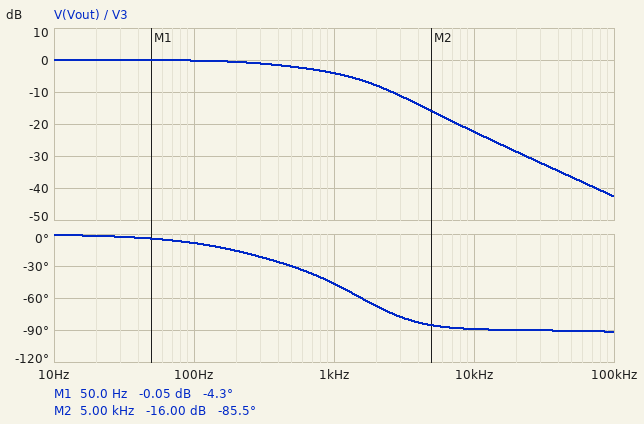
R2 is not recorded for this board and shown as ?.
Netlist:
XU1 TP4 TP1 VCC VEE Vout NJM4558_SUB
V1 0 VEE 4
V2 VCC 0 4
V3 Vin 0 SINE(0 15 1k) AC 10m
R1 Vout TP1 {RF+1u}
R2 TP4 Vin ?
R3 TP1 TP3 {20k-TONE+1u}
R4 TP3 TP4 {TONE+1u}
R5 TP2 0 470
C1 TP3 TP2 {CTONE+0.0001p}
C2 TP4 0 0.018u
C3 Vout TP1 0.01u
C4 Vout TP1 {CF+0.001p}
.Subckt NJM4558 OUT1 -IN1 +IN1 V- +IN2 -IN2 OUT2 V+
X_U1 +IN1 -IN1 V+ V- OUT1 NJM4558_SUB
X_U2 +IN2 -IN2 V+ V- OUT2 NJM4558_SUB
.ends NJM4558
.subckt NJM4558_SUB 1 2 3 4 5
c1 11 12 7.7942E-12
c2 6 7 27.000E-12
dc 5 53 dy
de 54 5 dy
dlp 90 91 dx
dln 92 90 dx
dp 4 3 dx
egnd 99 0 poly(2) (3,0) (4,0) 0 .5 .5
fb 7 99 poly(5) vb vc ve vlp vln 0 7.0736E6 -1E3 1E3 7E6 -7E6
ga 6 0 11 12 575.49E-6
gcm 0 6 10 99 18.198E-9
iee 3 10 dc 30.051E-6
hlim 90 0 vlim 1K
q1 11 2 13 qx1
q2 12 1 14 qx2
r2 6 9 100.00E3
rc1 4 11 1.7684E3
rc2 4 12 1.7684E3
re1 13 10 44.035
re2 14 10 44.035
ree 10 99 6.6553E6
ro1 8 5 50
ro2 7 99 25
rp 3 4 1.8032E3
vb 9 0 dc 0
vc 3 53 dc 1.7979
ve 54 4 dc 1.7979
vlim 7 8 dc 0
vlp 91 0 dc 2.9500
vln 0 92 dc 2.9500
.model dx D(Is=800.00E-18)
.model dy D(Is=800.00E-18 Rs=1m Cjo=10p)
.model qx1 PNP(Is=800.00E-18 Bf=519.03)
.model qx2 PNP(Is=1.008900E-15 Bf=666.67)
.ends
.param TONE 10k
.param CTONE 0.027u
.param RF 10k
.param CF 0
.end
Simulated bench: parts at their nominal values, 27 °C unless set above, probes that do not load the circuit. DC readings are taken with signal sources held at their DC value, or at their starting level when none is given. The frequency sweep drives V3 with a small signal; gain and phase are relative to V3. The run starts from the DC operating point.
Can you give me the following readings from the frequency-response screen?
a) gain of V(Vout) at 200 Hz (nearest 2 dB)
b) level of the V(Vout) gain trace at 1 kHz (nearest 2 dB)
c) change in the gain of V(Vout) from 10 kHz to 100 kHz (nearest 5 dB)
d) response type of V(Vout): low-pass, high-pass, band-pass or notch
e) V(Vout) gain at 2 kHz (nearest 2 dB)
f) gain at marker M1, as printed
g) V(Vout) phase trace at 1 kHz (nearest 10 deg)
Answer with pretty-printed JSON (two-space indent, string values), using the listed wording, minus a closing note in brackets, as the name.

{
  "gain of V(Vout) at 200 Hz": "0 dB",
  "level of the V(Vout) gain trace at 1 kHz": "-4 dB",
  "change in the gain of V(Vout) from 10 kHz to 100 kHz": "-20 dB",
  "response type of V(Vout): low-pass, high-pass, band-pass or notch": "low-pass",
  "V(Vout) gain at 2 kHz": "-8 dB",
  "gain at marker M1, as printed": "-0.05 dB",
  "V(Vout) phase trace at 1 kHz": "-50 deg"
}
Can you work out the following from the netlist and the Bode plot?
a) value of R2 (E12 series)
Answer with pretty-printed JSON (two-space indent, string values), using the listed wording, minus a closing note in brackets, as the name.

{
  "value of R2": "12 kΩ"
}
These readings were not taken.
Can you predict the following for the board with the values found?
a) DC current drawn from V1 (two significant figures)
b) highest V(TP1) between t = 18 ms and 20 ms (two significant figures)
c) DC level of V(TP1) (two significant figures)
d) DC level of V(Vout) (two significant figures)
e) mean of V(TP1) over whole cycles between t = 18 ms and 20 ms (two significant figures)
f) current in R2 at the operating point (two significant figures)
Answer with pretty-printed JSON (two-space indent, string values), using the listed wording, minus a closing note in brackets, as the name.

{
  "DC current drawn from V1": "4.5 mA",
  "highest V(TP1) between t = 18 ms and 20 ms": "4.4 V",
  "DC level of V(TP1)": "-9.4 mV",
  "DC level of V(Vout)": "-13 mV",
  "mean of V(TP1) over whole cycles between t = 18 ms and 20 ms": "790 mV",
  "current in R2 at the operating point": "280 nA"
}
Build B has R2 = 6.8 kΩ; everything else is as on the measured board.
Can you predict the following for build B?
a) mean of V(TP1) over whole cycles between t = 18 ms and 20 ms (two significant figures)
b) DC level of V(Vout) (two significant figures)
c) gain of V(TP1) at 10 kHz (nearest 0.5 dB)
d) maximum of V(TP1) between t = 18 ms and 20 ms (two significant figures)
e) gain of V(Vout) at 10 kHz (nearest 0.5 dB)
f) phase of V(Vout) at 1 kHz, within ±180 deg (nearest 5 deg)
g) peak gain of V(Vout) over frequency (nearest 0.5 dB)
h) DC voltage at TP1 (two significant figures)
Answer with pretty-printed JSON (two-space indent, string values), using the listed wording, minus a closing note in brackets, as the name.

{
  "mean of V(TP1) over whole cycles between t = 18 ms and 20 ms": "1.4 V",
  "DC level of V(Vout)": "-11 mV",
  "gain of V(TP1) at 10 kHz": "-18.0 dB",
  "maximum of V(TP1) between t = 18 ms and 20 ms": "5.0 V",
  "gain of V(Vout) at 10 kHz": "-17.5 dB",
  "phase of V(Vout) at 1 kHz, within ±180 deg": "-35 deg",
  "peak gain of V(Vout) over frequency": "0 dB",
  "DC voltage at TP1": "-7.9 mV"
}
